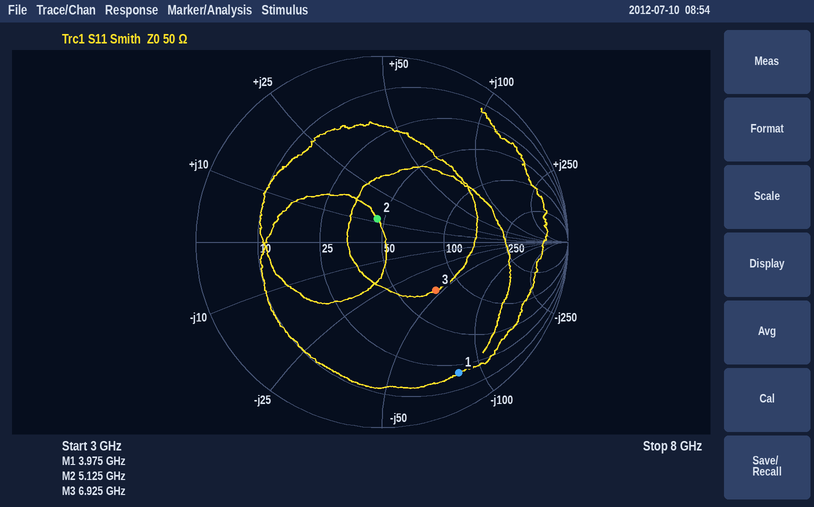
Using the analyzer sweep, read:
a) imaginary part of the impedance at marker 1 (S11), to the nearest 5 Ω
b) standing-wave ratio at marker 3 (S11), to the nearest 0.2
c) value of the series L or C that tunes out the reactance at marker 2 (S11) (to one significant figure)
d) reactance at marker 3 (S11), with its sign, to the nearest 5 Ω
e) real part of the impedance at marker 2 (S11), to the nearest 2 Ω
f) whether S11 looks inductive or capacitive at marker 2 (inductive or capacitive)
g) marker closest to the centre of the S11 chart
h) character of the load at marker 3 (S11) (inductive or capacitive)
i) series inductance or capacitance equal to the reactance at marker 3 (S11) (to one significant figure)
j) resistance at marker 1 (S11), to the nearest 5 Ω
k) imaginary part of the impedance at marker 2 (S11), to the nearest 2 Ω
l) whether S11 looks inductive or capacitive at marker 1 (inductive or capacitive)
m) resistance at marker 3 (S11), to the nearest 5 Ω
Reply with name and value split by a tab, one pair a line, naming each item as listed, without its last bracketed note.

imaginary part of the impedance at marker 1 (S11), to the nearest 5 Ω	-85 Ω
standing-wave ratio at marker 3 (S11), to the nearest 0.2	2.2
value of the series L or C that tunes out the reactance at marker 2 (S11)	3 pF
reactance at marker 3 (S11), with its sign, to the nearest 5 Ω	-45 Ω
real part of the impedance at marker 2 (S11), to the nearest 2 Ω	46 Ω
whether S11 looks inductive or capacitive at marker 2	inductive
marker closest to the centre of the S11 chart	marker 2
character of the load at marker 3 (S11)	capacitive
series inductance or capacitance equal to the reactance at marker 3 (S11)	500 fF
resistance at marker 1 (S11), to the nearest 5 Ω	20 Ω
imaginary part of the impedance at marker 2 (S11), to the nearest 2 Ω	+12 Ω
whether S11 looks inductive or capacitive at marker 1	capacitive
resistance at marker 3 (S11), to the nearest 5 Ω	75 Ω
